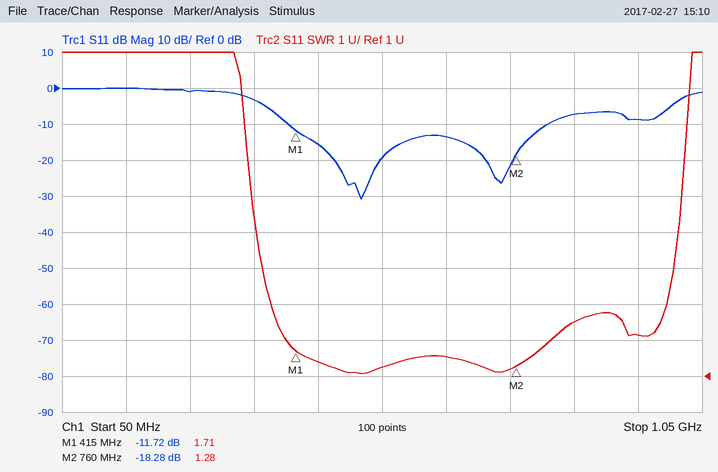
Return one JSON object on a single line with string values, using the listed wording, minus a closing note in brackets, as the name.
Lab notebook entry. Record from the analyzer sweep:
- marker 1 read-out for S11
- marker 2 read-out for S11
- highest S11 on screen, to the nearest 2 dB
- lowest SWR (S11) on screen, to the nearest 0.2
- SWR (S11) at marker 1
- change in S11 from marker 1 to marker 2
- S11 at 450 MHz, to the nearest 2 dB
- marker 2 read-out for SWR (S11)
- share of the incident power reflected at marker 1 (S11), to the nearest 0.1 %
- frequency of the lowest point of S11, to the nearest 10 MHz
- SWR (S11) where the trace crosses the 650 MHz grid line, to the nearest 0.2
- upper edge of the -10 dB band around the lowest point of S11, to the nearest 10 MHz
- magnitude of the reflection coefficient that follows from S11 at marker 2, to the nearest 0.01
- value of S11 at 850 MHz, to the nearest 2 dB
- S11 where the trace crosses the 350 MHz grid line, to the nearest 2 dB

{"marker 1 read-out for S11": "-11.72 dB", "marker 2 read-out for S11": "-18.28 dB", "highest S11 on screen, to the nearest 2 dB": "0 dB", "lowest SWR (S11) on screen, to the nearest 0.2": "1.0", "SWR (S11) at marker 1": "1.71", "change in S11 from marker 1 to marker 2": "-6.56 dB", "S11 at 450 MHz, to the nearest 2 dB": "-16 dB", "marker 2 read-out for SWR": "1.28", "share of the incident power reflected at marker 1 (S11), to the nearest 0.1 %": "6.7 %", "frequency of the lowest point of S11, to the nearest 10 MHz": "520 MHz", "SWR (S11) where the trace crosses the 650 MHz grid line, to the nearest 0.2": "1.6", "upper edge of the -10 dB band around the lowest point of S11, to the nearest 10 MHz": "810 MHz", "magnitude of the reflection coefficient that follows from S11 at marker 2, to the nearest 0.01": "0.12", "value of S11 at 850 MHz, to the nearest 2 dB": "-8 dB", "S11 where the trace crosses the 350 MHz grid line, to the nearest 2 dB": "-4 dB"}
